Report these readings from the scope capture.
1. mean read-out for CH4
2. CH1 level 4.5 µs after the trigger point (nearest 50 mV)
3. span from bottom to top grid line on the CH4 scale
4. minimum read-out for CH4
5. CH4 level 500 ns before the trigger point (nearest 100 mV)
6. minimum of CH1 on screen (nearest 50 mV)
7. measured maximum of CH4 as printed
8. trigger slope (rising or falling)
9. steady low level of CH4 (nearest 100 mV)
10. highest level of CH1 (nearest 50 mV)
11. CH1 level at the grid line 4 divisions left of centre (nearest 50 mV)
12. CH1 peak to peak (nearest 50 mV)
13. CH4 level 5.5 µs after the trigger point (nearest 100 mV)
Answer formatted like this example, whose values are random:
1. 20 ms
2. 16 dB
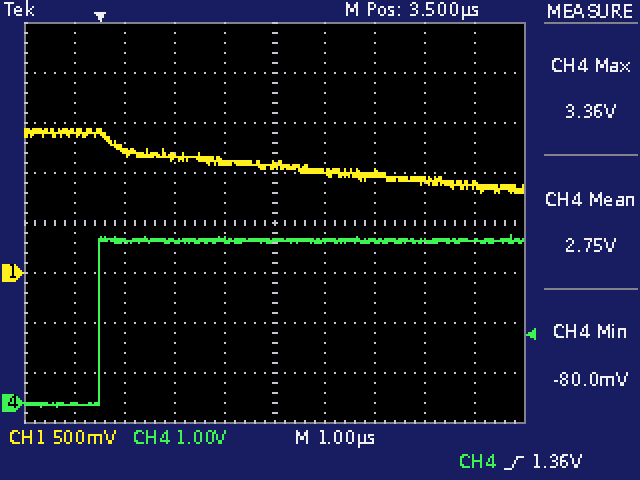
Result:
1. 2.75 V
2. 1.00 V
3. 8 V
4. -80.0 mV
5. 0.0 V
6. 800 mV
7. 3.36 V
8. rising
9. 0.0 V
10. 1.45 V
11. 1.40 V
12. 650 mV
13. 3.2 V
